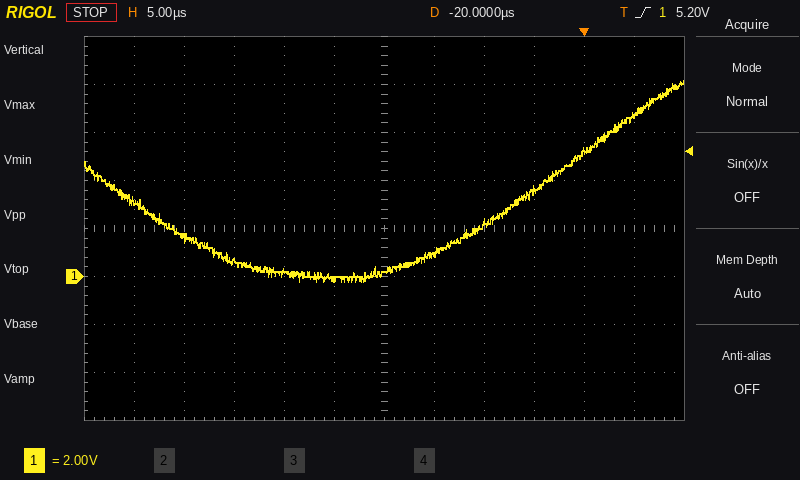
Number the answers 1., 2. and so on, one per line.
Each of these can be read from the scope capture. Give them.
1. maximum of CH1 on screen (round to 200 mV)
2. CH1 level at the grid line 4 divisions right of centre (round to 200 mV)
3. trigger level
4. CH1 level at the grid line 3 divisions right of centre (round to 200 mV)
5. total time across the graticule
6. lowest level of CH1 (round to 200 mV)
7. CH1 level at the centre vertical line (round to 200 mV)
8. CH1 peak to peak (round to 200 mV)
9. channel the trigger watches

1. 8.2 V
2. 5.2 V
3. 5.20 V
4. 3.6 V
5. 60 µs
6. -200 mV
7. 200 mV
8. 8.4 V
9. CH1
